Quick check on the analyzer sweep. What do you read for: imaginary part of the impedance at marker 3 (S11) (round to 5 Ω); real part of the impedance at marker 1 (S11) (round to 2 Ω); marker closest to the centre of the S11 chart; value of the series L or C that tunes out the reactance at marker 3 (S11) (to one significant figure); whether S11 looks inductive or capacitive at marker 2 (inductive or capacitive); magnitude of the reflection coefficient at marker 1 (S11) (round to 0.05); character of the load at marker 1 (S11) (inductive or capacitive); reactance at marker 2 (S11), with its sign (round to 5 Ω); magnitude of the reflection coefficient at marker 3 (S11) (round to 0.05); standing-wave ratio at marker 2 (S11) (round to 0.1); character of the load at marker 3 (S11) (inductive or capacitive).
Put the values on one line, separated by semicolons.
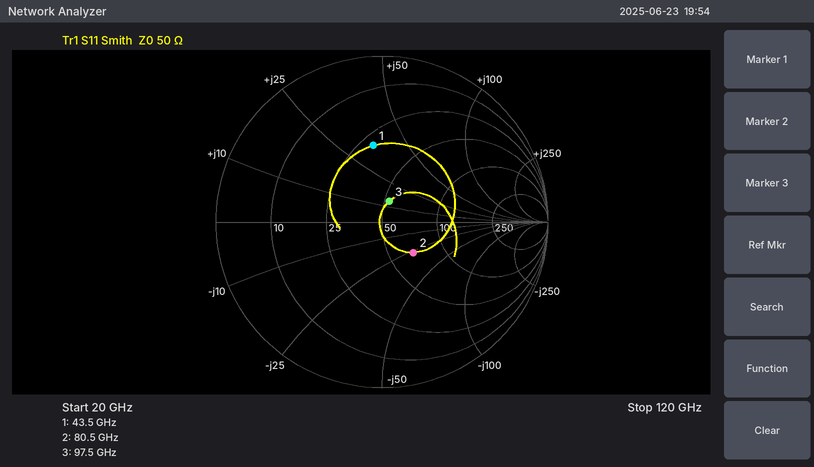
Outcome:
+15 Ω; 30 Ω; marker 3; 100 fF; capacitive; 0.45; inductive; -25 Ω; 0.15; 1.7; inductive
